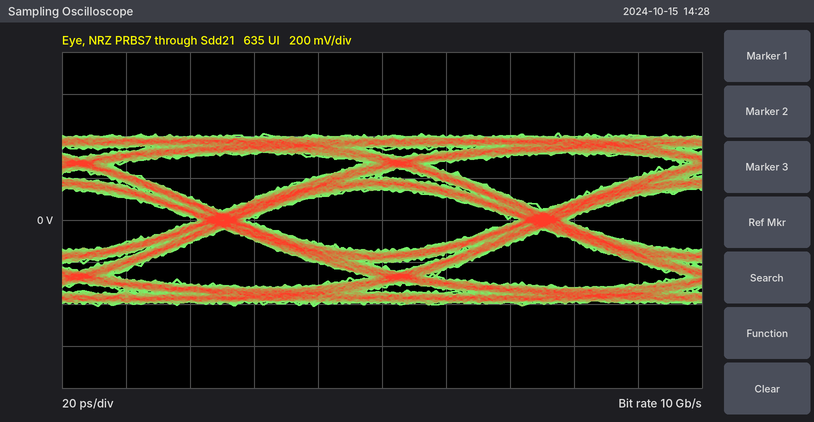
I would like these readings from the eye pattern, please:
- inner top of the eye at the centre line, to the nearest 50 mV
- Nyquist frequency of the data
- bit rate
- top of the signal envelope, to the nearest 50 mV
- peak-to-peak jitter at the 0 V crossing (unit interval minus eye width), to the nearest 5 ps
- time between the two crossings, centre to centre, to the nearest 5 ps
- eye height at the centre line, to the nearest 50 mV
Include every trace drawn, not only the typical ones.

150 mV
5 GHz
10 Gb/s
400 mV
15 ps
100 ps
300 mV
